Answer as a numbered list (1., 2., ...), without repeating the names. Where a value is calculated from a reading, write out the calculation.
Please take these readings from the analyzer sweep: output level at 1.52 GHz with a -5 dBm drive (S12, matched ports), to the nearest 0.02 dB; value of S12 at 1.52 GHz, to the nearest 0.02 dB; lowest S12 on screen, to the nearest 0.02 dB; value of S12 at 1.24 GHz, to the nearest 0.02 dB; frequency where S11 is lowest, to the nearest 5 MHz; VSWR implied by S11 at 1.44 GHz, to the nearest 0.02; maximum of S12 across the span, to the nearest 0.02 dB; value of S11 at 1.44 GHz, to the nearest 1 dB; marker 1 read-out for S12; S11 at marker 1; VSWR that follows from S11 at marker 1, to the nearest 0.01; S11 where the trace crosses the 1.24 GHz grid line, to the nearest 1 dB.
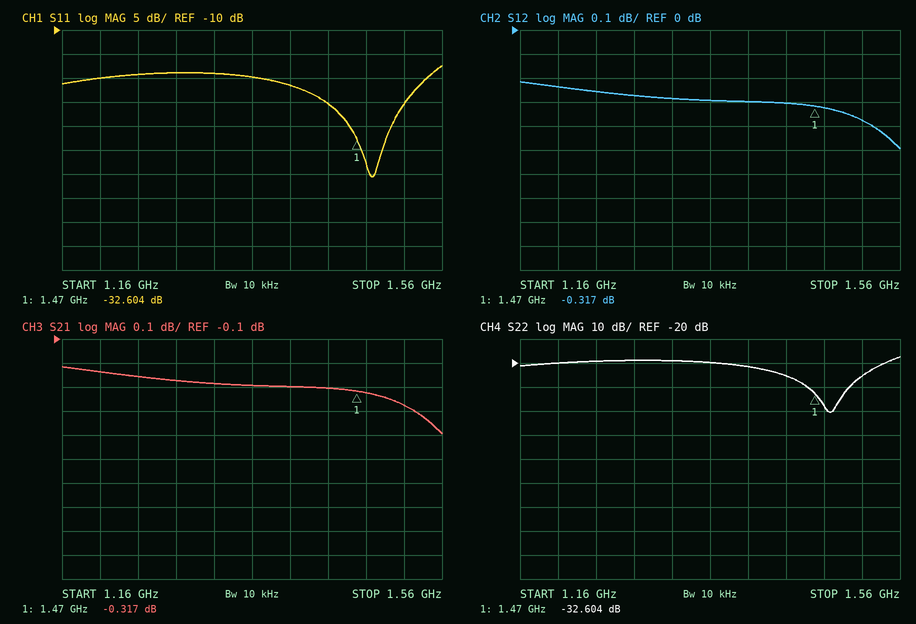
1. -5 dBm + (-0.38 dB) = -5.38 dBm
2. -0.38 dB
3. -0.50 dB
4. -0.26 dB
5. 1.485 GHz
6. |Γ| = 10^(-25/20) = 0.0562; VSWR = (1 + 0.0562)/(1 − 0.0562) ≈ 1.12
7. -0.22 dB
8. -25 dB
9. -0.317 dB
10. -32.604 dB
11. (1 + 0.0234)/(1 − 0.0234) ≈ 1.05
12. -19 dB
